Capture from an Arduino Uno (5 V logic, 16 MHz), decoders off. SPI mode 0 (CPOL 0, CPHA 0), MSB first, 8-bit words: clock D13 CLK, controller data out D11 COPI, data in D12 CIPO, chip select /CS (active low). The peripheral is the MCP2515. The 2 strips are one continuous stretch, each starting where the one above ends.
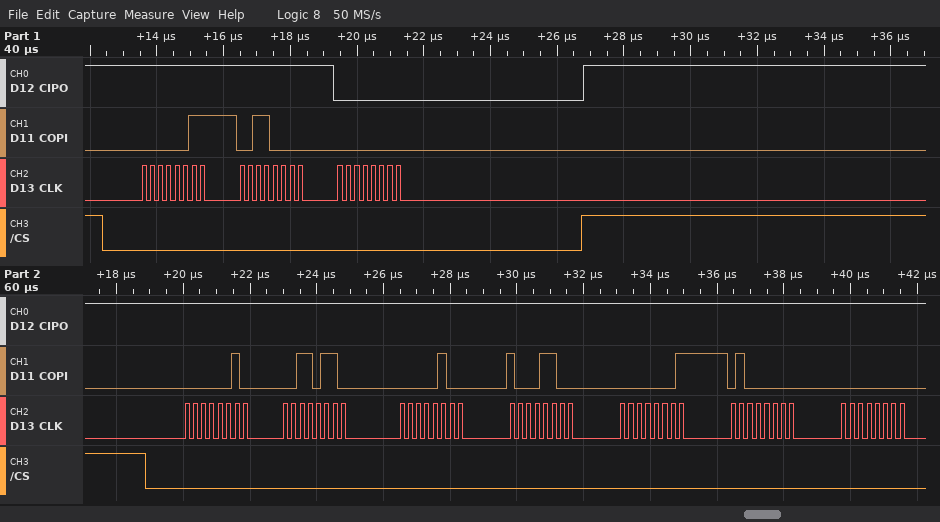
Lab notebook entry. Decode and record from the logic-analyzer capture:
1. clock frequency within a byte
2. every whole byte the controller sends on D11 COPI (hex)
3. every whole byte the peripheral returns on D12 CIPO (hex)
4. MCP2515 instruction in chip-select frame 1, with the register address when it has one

4 MHz
03 30 00 02 36 04 8C 01 40 00
FF FF 00 FF FF FF FF FF FF FF
READ 0x30
